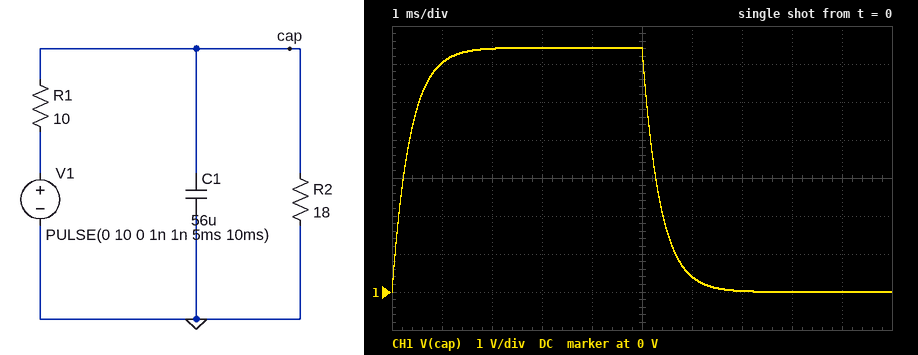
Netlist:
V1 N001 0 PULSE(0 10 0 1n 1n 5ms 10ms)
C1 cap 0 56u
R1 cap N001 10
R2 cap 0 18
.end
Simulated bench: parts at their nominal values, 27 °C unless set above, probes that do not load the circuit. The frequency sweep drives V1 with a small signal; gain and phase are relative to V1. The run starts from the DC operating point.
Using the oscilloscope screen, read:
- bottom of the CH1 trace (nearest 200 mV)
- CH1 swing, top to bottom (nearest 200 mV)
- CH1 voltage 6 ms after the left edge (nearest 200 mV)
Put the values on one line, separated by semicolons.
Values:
0 V; 6.4 V; 400 mV
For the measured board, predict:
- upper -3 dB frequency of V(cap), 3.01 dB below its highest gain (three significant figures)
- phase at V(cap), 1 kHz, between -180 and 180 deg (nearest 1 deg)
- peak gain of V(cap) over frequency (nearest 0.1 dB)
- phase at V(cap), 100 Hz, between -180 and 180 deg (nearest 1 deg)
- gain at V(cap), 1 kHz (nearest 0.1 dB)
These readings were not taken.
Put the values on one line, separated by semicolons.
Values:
442 Hz; -66 deg; -3.8 dB; -13 deg; -11.7 dB
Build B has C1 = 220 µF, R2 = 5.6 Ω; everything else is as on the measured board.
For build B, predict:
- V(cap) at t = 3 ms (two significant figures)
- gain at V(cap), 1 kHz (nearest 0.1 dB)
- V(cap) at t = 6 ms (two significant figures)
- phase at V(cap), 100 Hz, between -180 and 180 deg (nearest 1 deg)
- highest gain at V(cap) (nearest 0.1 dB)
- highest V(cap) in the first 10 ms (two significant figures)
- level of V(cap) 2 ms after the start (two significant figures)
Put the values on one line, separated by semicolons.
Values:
3.5 V; -23.0 dB; 1.0 V; -26 deg; -8.9 dB; 3.6 V; 3.3 V
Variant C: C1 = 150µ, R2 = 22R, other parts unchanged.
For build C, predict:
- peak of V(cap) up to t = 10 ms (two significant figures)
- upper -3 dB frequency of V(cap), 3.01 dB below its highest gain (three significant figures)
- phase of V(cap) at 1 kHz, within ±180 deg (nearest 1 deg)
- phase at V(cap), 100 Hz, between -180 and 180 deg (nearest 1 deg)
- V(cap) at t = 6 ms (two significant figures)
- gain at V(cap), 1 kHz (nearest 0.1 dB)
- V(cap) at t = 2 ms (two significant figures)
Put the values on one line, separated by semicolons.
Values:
6.8 V; 154 Hz; -81 deg; -33 deg; 2.6 V; -19.6 dB; 5.9 V
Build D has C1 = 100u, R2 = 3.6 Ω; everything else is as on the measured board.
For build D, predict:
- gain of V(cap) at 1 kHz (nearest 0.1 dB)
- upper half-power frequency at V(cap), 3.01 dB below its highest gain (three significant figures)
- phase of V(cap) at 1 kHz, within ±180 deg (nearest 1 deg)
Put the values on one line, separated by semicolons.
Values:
-17.3 dB; 601 Hz; -59 deg
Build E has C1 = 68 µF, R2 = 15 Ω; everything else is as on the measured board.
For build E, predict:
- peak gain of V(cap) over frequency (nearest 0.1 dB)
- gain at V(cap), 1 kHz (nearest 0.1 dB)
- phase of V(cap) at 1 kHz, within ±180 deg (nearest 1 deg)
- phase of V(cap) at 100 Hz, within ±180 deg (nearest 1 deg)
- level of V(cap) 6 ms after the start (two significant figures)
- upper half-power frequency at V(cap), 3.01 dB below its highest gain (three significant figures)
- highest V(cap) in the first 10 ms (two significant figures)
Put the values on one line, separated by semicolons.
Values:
-4.4 dB; -13.2 dB; -69 deg; -14 deg; 520 mV; 390 Hz; 6.0 V
